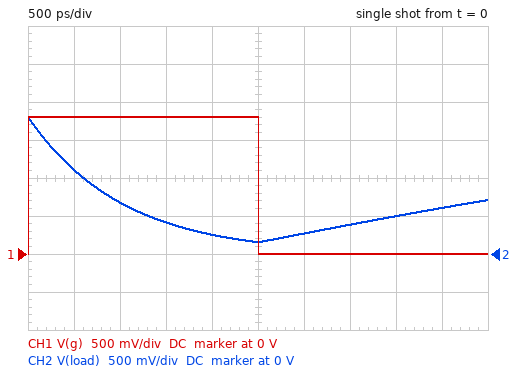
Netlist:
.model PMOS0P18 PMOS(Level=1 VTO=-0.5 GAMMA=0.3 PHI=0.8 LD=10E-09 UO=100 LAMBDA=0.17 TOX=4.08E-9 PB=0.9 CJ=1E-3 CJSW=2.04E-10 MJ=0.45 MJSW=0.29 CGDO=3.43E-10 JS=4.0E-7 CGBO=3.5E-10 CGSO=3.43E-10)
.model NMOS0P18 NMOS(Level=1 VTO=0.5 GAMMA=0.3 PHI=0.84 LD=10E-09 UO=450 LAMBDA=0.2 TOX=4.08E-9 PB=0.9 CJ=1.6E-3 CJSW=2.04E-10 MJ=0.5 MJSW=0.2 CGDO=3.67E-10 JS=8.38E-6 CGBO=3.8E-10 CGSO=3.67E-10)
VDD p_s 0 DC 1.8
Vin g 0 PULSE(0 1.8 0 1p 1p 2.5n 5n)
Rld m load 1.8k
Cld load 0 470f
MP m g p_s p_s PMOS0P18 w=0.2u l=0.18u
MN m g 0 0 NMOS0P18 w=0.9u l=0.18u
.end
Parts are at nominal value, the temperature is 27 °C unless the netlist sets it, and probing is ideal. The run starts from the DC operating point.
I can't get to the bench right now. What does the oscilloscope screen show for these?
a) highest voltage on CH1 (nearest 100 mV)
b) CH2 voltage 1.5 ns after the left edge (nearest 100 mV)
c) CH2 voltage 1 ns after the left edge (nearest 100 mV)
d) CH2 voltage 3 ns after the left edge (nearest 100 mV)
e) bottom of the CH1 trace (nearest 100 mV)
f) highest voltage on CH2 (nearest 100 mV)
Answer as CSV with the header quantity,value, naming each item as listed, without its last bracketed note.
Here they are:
quantity,value
highest voltage on CH1,1.8 V
CH2 voltage 1.5 ns after the left edge,400 mV
CH2 voltage 1 ns after the left edge,700 mV
CH2 voltage 3 ns after the left edge,300 mV
bottom of the CH1 trace,0 V
highest voltage on CH2,1.8 V
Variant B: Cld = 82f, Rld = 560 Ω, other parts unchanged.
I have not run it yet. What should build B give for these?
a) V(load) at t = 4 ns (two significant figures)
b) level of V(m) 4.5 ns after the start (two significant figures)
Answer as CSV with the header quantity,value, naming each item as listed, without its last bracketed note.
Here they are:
quantity,value
V(load) at t = 4 ns,1.5 V
level of V(m) 4.5 ns after the start,1.7 V
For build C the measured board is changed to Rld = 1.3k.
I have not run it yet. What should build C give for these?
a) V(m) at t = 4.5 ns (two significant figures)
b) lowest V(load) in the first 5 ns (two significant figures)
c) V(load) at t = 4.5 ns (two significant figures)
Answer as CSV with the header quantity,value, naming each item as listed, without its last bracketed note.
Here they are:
quantity,value
V(m) at t = 4.5 ns,670 mV
lowest V(load) in the first 5 ns,73 mV
V(load) at t = 4.5 ns,540 mV
